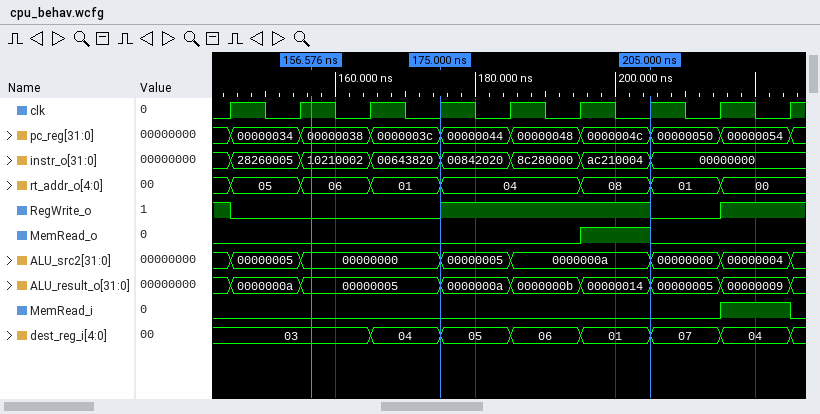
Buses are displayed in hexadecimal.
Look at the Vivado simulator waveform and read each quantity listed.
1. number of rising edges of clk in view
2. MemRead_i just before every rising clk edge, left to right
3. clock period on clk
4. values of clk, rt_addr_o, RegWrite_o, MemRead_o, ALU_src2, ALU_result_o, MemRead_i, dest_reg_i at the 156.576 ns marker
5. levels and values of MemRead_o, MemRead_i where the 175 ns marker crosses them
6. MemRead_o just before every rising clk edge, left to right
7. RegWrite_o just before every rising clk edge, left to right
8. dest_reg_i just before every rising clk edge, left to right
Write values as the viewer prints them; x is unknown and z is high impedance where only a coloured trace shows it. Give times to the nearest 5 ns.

9
0 0 0 0 0 0 0 0 1
10 ns
clk=1, rt_addr_o=06, RegWrite_o=0, MemRead_o=0, ALU_src2=00000000, ALU_result_o=00000005, MemRead_i=0, dest_reg_i=03
MemRead_o=0, MemRead_i=0
0 0 0 0 0 0 1 0 0
1 0 0 0 1 1 1 0 1
03, 03, 03, 04, 05, 06, 01, 07, 04
